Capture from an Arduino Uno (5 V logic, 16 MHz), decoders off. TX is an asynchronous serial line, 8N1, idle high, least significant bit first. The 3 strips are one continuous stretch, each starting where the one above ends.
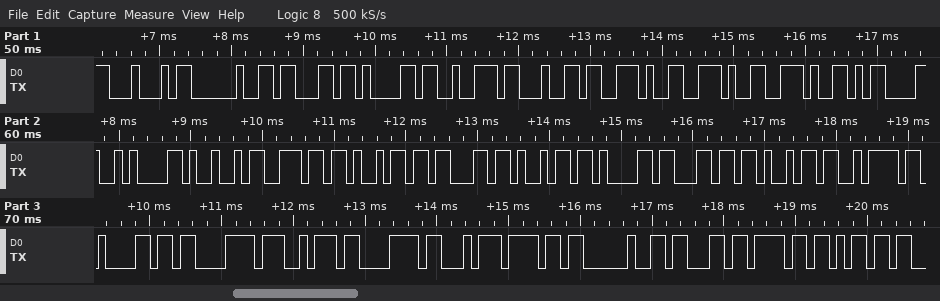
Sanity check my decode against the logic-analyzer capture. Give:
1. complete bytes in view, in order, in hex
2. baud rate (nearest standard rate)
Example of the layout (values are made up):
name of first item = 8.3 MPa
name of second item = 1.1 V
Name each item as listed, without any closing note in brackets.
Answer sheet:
complete bytes in view, in order, in hex = 44 20 63 61 72 64 2E 2E 2E 0D 0A 49 6E 69 63 69 61 6C 69 7A 61 C3 A7 C3 A3 6F 20 63 6F 6D
baud rate = 9600 baud
